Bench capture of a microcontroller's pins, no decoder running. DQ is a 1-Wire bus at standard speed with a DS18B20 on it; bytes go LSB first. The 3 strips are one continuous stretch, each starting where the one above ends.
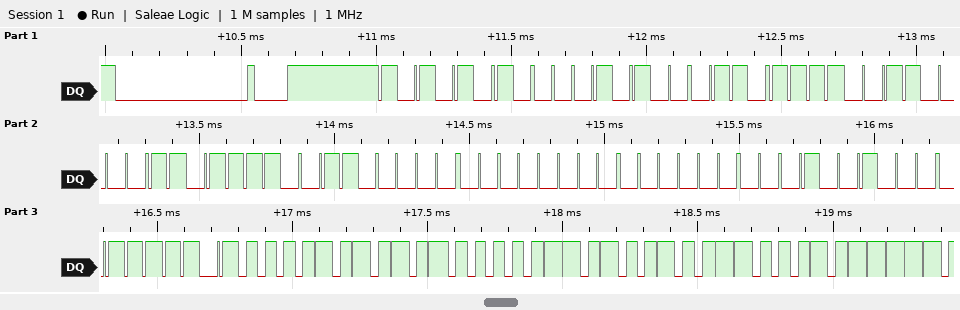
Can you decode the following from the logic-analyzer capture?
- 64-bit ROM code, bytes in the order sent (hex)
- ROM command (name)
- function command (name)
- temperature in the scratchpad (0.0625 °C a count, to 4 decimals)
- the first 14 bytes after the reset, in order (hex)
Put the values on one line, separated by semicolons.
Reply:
28 F6 0C 7B 06 00 00 12; Match ROM; Read Scratchpad; 85.0000 °C; 55 28 F6 0C 7B 06 00 00 12 BE 50 05 4B 46
